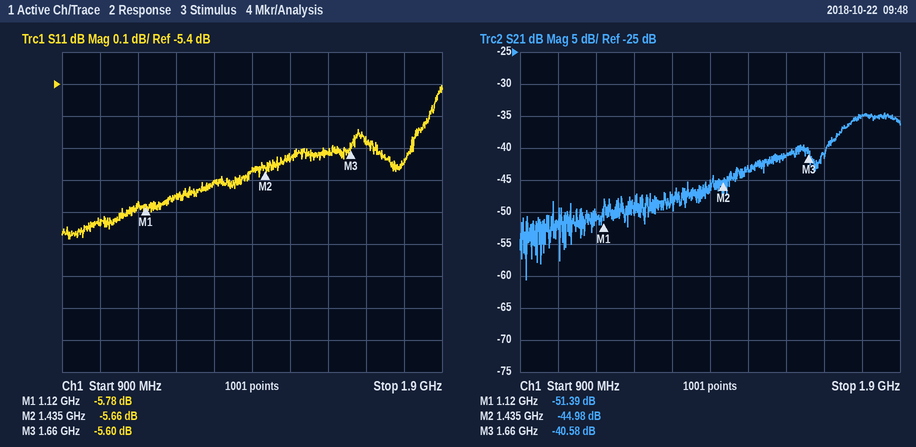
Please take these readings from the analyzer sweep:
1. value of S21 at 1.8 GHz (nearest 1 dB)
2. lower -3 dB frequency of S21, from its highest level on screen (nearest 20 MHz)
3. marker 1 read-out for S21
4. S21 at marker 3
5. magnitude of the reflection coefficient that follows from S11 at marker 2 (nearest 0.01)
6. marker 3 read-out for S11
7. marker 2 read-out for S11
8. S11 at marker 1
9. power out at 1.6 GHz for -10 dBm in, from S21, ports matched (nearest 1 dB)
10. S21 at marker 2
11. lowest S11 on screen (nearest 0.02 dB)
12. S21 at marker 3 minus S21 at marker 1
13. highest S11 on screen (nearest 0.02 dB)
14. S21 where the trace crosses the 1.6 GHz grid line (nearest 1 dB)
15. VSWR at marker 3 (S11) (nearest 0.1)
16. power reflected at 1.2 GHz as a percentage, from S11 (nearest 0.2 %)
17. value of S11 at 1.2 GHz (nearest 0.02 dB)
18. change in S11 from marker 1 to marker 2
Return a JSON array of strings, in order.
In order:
["-35 dB", "1.74 GHz", "-51.39 dB", "-40.58 dB", "0.52", "-5.60 dB", "-5.66 dB", "-5.78 dB", "-51 dBm", "-44.98 dB", "-5.88 dB", "10.81 dB", "-5.40 dB", "-41 dB", "3.2", "26.6 %", "-5.76 dB", "0.12 dB"]
